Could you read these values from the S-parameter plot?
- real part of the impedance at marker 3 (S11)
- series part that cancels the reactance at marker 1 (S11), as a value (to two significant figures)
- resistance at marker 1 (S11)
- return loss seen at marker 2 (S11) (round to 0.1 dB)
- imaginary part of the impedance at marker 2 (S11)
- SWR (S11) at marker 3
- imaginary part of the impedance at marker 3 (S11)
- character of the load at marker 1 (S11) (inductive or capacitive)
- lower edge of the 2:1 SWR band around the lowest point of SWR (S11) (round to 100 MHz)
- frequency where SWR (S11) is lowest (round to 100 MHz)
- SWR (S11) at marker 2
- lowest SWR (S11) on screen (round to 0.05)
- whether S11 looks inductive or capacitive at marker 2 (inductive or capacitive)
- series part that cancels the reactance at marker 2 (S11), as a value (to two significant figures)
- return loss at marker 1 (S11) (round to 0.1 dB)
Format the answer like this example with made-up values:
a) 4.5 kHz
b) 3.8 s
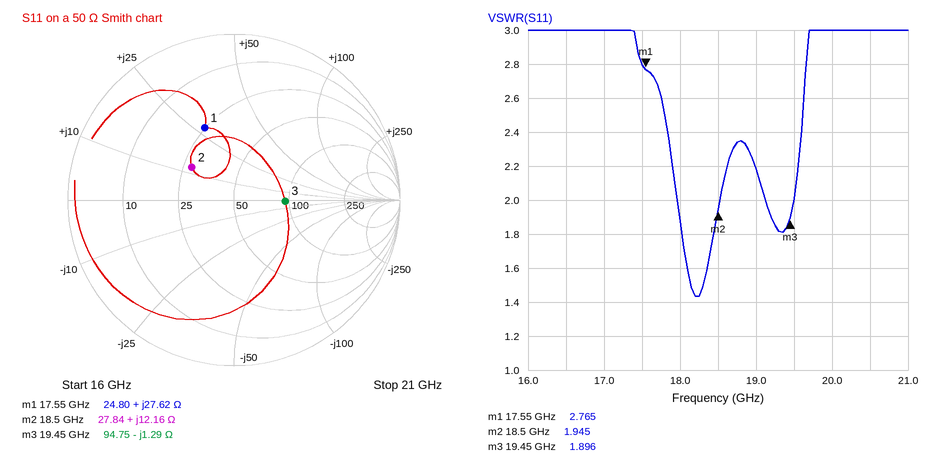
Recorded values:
a) 94.75 Ω
b) 330 fF
c) 24.80 Ω
d) 9.9 dB
e) +12.16 Ω
f) 1.896
g) -1.29 Ω
h) inductive
i) 18.0 GHz
j) 18.2 GHz
k) 1.945
l) 1.45
m) inductive
n) 710 fF
o) 6.6 dB
